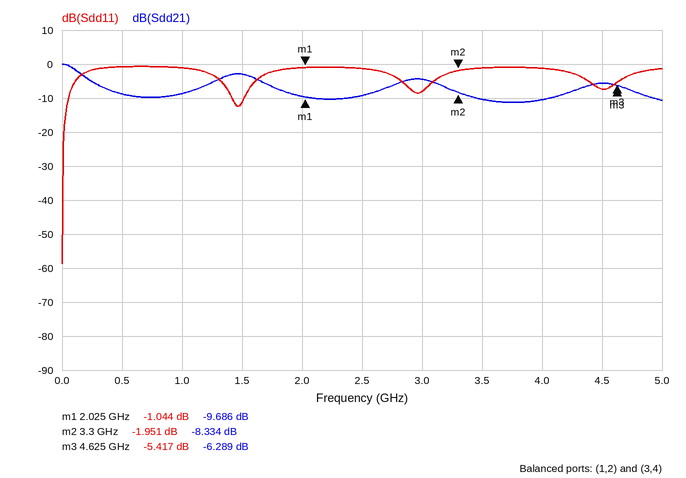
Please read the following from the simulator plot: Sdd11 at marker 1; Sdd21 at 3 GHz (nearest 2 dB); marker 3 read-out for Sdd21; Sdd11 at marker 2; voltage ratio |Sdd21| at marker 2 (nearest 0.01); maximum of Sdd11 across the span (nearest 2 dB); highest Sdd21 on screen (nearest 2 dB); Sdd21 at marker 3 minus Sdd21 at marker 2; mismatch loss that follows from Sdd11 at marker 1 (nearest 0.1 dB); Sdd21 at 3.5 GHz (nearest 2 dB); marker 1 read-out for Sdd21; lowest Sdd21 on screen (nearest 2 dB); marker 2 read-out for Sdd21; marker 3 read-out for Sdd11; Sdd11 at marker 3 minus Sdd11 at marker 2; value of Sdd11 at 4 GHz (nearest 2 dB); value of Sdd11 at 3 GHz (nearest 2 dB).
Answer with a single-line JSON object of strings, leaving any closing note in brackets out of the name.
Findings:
{"Sdd11 at marker 1": "-1.044 dB", "Sdd21 at 3 GHz": "-4 dB", "marker 3 read-out for Sdd21": "-6.289 dB", "Sdd11 at marker 2": "-1.951 dB", "voltage ratio |Sdd21| at marker 2": "0.38", "maximum of Sdd11 across the span": "0 dB", "highest Sdd21 on screen": "0 dB", "Sdd21 at marker 3 minus Sdd21 at marker 2": "2.045 dB", "mismatch loss that follows from Sdd11 at marker 1": "6.7 dB", "Sdd21 at 3.5 GHz": "-10 dB", "marker 1 read-out for Sdd21": "-9.686 dB", "lowest Sdd21 on screen": "-12 dB", "marker 2 read-out for Sdd21": "-8.334 dB", "marker 3 read-out for Sdd11": "-5.417 dB", "Sdd11 at marker 3 minus Sdd11 at marker 2": "-3.466 dB", "value of Sdd11 at 4 GHz": "-2 dB", "value of Sdd11 at 3 GHz": "-8 dB"}
